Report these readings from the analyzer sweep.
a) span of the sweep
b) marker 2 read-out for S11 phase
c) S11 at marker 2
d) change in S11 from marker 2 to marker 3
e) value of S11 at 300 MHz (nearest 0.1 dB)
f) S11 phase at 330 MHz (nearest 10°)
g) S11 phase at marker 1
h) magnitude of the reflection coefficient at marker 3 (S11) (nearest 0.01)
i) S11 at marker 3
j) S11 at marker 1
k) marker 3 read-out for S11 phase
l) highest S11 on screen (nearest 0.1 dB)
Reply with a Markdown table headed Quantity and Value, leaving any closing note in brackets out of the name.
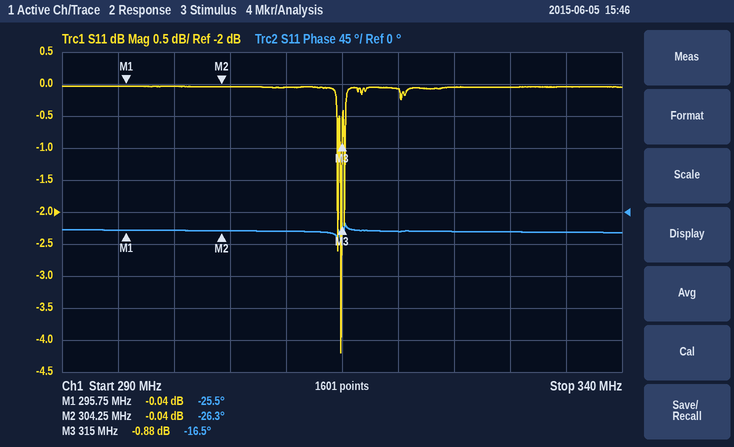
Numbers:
| Quantity | Value |
|---|---|
| span of the sweep | 50 MHz |
| marker 2 read-out for S11 phase | -26.3° |
| S11 at marker 2 | -0.04 dB |
| change in S11 from marker 2 to marker 3 | -0.84 dB |
| value of S11 at 300 MHz | 0.0 dB |
| S11 phase at 330 MHz | -30° |
| S11 phase at marker 1 | -25.5° |
| magnitude of the reflection coefficient at marker 3 (S11) | 0.90 |
| S11 at marker 3 | -0.88 dB |
| S11 at marker 1 | -0.04 dB |
| marker 3 read-out for S11 phase | -16.5° |
| highest S11 on screen | 0.0 dB |
